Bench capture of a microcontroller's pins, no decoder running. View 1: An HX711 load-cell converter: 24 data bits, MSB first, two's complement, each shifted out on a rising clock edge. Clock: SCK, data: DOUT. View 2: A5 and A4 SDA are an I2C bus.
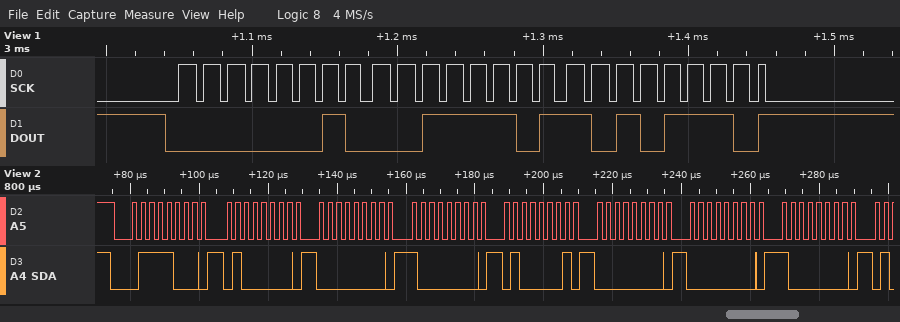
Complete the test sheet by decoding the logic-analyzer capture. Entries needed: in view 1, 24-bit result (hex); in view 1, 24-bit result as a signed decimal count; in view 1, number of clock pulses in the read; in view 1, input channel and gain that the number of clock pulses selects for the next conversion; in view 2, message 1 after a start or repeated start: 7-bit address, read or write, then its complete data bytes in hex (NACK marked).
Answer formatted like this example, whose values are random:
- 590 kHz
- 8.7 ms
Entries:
- 0x023DAE
- 146862
- 25
- channel A, gain 128
- 0x3C write: 40 00 80 41 00 00 80
